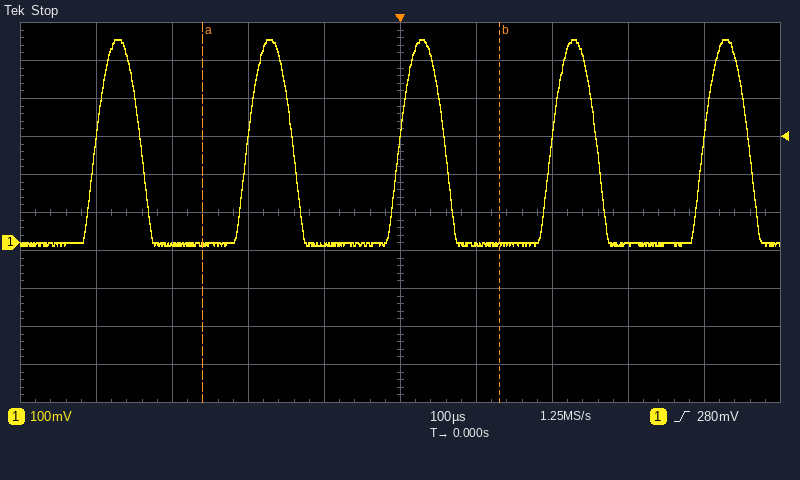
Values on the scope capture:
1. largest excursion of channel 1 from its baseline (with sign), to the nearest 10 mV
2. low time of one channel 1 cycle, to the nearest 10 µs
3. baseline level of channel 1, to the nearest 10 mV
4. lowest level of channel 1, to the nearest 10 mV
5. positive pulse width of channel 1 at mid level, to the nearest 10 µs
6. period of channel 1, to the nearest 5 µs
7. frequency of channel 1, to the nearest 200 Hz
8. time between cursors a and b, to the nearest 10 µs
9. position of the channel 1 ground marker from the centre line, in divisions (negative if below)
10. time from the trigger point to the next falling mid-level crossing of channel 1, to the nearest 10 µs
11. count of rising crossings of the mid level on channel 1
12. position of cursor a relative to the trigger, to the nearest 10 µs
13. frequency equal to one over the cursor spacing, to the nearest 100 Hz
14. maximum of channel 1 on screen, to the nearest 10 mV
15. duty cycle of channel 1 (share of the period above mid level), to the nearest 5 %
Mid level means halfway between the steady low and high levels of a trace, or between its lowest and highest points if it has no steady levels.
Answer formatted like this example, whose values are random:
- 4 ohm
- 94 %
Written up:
- +540 mV
- 140 µs
- 0 mV
- -10 mV
- 60 µs
- 200 µs
- 5.0 kHz
- 390 µs
- -0.8 div
- 60 µs
- 5
- -260 µs
- 2.6 kHz
- 540 mV
- 30 %
